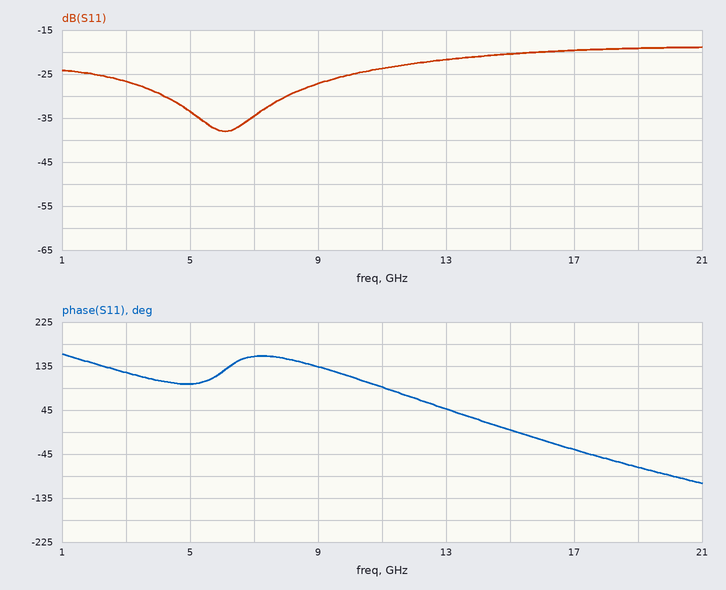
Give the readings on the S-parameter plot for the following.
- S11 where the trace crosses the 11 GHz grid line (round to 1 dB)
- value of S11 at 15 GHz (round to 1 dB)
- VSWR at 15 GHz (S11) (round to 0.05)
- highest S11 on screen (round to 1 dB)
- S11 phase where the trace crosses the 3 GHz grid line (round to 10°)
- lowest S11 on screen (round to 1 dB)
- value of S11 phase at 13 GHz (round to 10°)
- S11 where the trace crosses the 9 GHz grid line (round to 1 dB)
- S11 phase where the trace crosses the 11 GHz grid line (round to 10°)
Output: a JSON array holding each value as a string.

["-24 dB", "-20 dB", "1.20", "-19 dB", "120°", "-38 dB", "50°", "-27 dB", "90°"]
